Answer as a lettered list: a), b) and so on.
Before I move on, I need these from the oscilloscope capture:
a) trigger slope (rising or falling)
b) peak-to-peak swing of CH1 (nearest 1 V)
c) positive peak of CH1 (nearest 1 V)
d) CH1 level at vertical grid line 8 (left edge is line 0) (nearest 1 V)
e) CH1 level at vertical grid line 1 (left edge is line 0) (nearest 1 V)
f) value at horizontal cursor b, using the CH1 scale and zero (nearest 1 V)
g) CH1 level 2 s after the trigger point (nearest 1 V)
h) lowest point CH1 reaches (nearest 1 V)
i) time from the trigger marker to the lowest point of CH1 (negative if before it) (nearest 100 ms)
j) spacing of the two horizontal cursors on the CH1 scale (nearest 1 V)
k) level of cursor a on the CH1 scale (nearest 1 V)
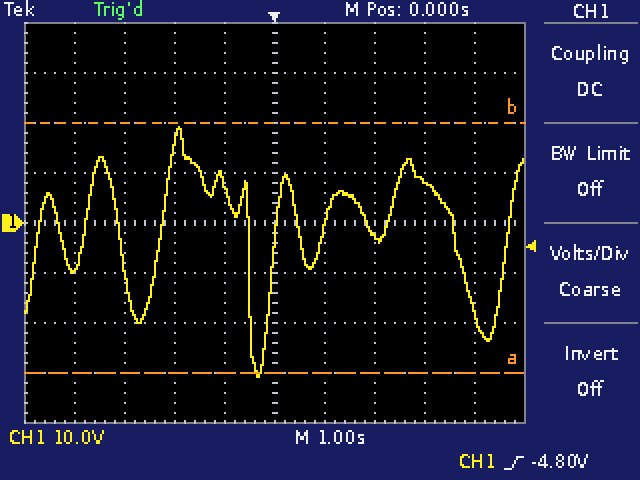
a) rising
b) 50 V
c) 19 V
d) 8 V
e) -9 V
f) 20 V
g) -2 V
h) -31 V
i) -300 ms
j) 50 V
k) -30 V
